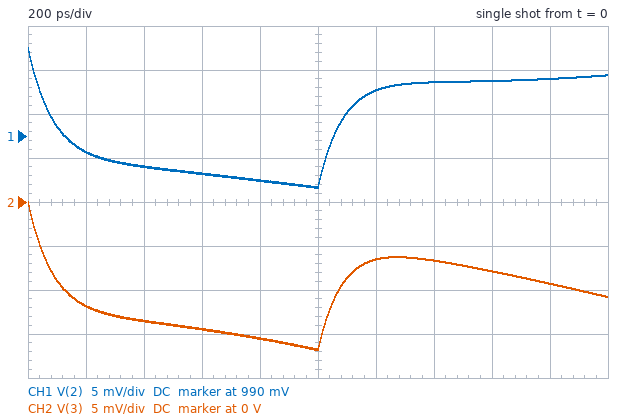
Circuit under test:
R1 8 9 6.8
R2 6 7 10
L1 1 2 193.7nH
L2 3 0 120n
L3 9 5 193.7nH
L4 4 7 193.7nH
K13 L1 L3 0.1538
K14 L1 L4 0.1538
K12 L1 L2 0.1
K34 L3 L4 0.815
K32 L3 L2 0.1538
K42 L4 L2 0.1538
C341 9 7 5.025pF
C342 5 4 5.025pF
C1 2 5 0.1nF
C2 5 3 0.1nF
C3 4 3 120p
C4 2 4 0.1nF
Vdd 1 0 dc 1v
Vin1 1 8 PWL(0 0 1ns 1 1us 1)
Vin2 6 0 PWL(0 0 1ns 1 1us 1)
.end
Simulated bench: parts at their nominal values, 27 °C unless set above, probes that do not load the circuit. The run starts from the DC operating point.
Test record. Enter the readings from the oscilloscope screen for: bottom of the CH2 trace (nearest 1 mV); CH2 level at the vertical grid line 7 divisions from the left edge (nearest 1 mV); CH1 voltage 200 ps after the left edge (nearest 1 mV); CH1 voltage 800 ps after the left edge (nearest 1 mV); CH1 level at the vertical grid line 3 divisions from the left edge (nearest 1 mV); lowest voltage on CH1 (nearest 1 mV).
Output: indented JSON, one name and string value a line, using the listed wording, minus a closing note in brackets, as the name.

{
  "bottom of the CH2 trace": "-17 mV",
  "CH2 level at the vertical grid line 7 divisions from the left edge": "-7 mV",
  "CH1 voltage 200 ps after the left edge": "988 mV",
  "CH1 voltage 800 ps after the left edge": "985 mV",
  "CH1 level at the vertical grid line 3 divisions from the left edge": "986 mV",
  "lowest voltage on CH1": "984 mV"
}
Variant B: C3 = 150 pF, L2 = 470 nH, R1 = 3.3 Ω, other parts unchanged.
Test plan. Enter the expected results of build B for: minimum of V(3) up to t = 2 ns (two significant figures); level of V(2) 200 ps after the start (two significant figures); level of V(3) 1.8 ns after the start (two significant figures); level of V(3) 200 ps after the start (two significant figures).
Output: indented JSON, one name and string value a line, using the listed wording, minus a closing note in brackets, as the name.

{
  "minimum of V(3) up to t = 2 ns": "-28 mV",
  "level of V(2) 200 ps after the start": "970 mV",
  "level of V(3) 1.8 ns after the start": "-3.6 mV",
  "level of V(3) 200 ps after the start": "-27 mV"
}
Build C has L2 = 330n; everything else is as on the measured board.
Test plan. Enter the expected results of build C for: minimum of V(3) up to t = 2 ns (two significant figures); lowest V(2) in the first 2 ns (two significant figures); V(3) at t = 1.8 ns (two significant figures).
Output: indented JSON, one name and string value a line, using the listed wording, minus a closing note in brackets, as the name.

{
  "minimum of V(3) up to t = 2 ns": "-13 mV",
  "lowest V(2) in the first 2 ns": "990 mV",
  "V(3) at t = 1.8 ns": "-1.8 mV"
}
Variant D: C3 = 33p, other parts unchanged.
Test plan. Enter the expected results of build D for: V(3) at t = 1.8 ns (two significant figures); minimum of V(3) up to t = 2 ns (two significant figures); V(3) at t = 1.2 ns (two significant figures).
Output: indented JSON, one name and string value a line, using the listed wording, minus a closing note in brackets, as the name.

{
  "V(3) at t = 1.8 ns": "-18 mV",
  "minimum of V(3) up to t = 2 ns": "-23 mV",
  "V(3) at t = 1.2 ns": "-9.2 mV"
}
